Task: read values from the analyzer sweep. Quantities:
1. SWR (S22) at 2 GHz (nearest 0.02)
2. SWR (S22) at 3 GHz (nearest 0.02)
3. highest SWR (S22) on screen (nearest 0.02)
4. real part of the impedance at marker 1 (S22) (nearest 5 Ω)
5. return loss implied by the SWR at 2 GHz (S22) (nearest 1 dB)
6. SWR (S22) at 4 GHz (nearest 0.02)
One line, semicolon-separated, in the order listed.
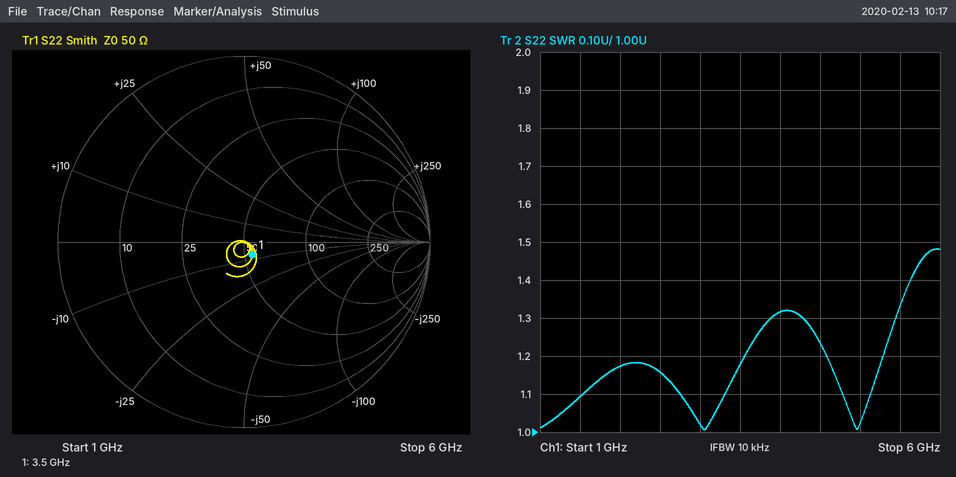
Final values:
1.18; 1.02; 1.48; 55 Ω; 22 dB; 1.32
